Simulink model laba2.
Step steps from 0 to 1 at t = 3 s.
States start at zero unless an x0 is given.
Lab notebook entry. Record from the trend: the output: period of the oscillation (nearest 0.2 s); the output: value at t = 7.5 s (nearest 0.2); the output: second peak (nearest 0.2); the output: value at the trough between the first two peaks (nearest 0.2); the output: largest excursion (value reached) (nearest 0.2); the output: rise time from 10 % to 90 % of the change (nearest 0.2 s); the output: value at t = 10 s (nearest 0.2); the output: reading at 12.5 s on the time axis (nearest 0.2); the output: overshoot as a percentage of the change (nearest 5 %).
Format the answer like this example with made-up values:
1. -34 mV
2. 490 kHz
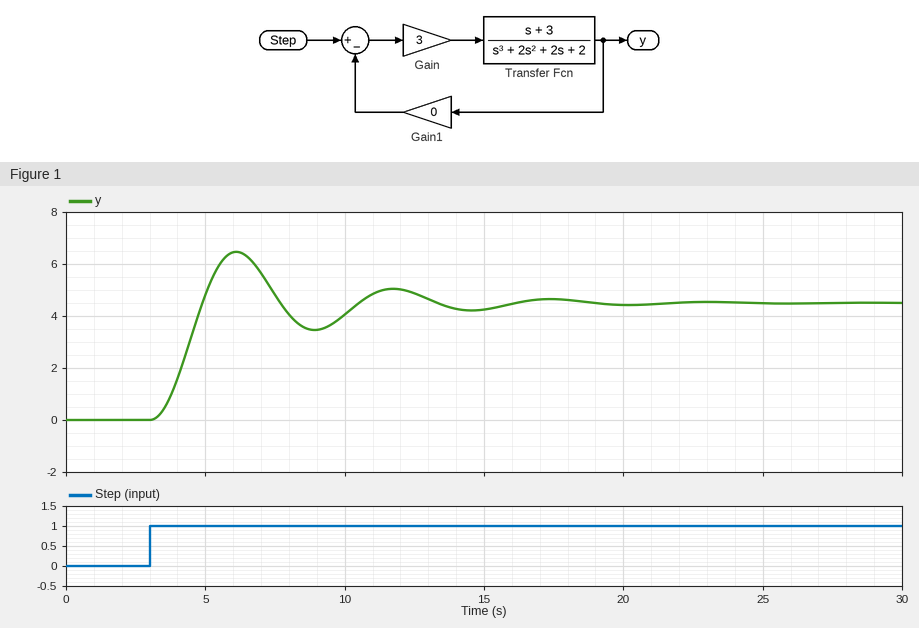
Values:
1. 5.6 s
2. 4.8
3. 5.0
4. 3.4
5. 6.4
6. 1.2 s
7. 4.0
8. 4.8
9. 45 %
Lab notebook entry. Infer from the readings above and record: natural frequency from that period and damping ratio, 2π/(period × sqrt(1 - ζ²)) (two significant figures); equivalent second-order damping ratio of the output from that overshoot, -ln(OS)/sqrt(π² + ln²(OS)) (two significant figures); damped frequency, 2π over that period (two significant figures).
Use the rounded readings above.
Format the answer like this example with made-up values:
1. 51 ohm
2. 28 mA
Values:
1. 1.2 rad/s
2. 0.25
3. 1.1 rad/s
